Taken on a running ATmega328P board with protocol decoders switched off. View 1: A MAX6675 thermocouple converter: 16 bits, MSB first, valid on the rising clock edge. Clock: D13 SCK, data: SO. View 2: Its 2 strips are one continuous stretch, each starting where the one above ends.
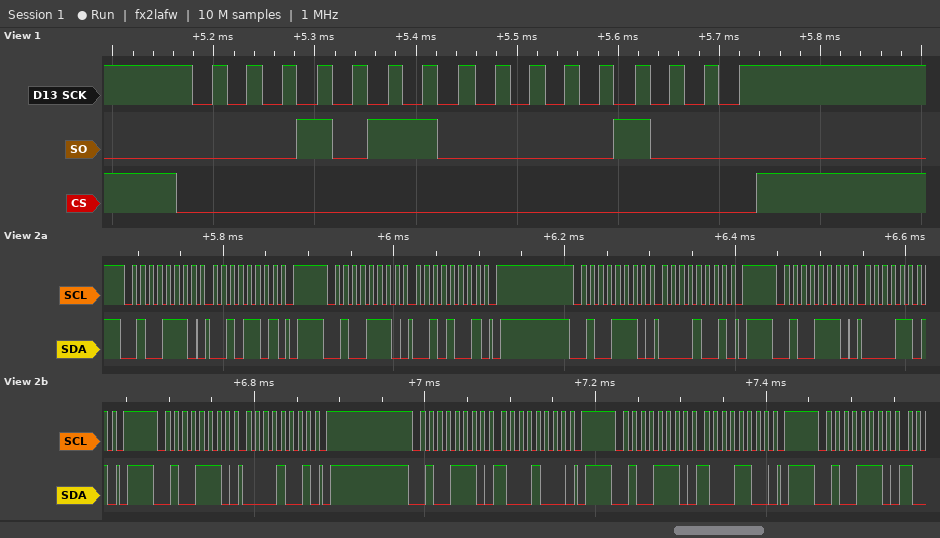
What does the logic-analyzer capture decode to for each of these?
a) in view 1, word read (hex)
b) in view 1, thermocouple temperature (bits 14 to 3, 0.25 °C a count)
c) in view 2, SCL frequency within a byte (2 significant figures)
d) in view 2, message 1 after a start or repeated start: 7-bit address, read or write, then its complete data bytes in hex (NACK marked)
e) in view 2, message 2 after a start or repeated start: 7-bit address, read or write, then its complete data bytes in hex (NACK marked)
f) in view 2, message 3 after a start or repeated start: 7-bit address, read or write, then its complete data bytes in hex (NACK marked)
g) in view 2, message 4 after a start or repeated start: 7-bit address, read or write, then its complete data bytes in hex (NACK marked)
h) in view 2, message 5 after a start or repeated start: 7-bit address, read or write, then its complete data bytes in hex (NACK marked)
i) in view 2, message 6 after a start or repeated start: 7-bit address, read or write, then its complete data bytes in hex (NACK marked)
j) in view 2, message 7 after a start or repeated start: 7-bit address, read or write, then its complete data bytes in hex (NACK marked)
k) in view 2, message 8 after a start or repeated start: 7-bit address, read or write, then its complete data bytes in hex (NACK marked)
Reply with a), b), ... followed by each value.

a) 0x1608
b) 176.25 °C
c) 100 kHz
d) 0x27 write: 2D
e) 0x27 write: 29
f) 0x27 write: 09
g) 0x27 write: 0D
h) 0x27 write: 09
i) 0x27 write: 88
j) 0x27 write: 8C
k) 0x27 write
